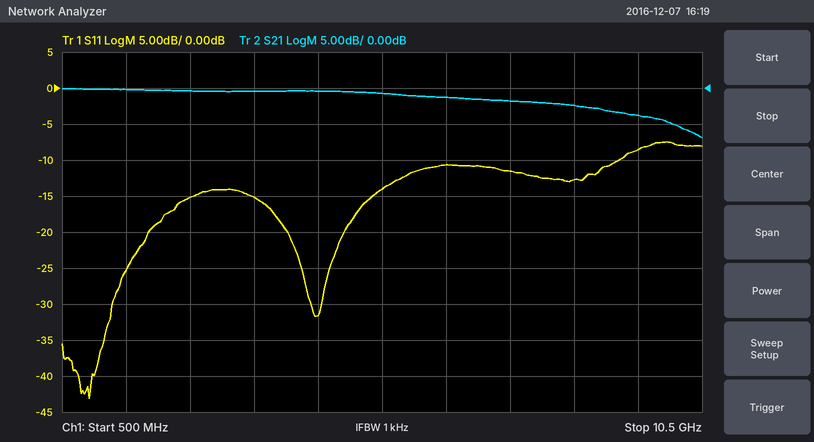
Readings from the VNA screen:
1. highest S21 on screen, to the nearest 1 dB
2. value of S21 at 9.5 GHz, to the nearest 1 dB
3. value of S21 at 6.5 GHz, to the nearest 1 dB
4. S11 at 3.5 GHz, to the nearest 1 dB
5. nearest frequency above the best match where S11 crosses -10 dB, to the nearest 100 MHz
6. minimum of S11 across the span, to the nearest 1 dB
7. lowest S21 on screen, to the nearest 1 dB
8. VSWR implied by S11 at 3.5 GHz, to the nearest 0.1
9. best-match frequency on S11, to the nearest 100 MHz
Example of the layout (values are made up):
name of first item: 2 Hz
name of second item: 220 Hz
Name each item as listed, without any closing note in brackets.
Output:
highest S21 on screen, to the nearest 1 dB: 0 dB
value of S21 at 9.5 GHz, to the nearest 1 dB: -4 dB
value of S21 at 6.5 GHz, to the nearest 1 dB: -1 dB
S11 at 3.5 GHz, to the nearest 1 dB: -15 dB
nearest frequency above the best match where S11 crosses -10 dB, to the nearest 100 MHz: 9.2 GHz
minimum of S11 across the span, to the nearest 1 dB: -43 dB
lowest S21 on screen, to the nearest 1 dB: -7 dB
VSWR implied by S11 at 3.5 GHz, to the nearest 0.1: 1.4
best-match frequency on S11, to the nearest 100 MHz: 900 MHz
